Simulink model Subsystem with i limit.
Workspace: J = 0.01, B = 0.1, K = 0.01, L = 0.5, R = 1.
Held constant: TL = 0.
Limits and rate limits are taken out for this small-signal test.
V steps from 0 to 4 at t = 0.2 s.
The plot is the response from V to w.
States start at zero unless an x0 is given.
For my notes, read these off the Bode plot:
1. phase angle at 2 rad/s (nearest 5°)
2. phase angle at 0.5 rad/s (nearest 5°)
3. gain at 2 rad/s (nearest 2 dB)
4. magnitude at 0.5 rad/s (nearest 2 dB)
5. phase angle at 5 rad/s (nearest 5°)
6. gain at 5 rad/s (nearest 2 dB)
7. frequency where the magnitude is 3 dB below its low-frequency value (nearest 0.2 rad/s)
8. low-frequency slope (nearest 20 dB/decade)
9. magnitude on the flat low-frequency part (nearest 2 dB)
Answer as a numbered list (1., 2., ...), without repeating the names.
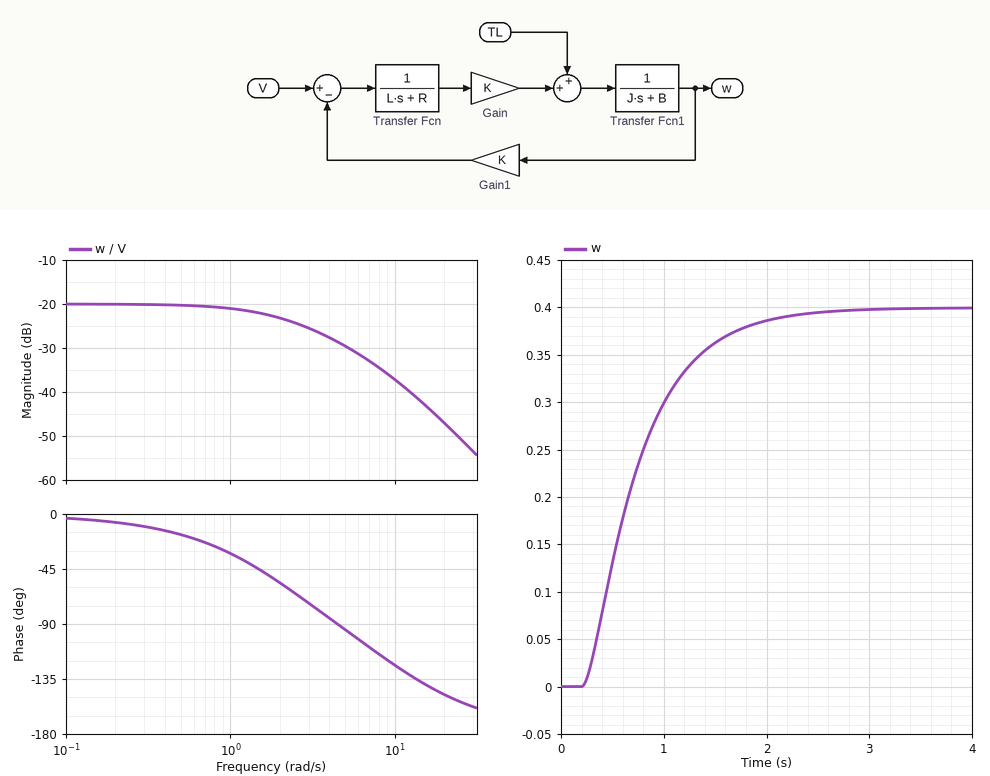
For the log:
1. -55°
2. -15°
3. -24 dB
4. -20 dB
5. -95°
6. -30 dB
7. 2.0 rad/s
8. 0 dB/decade
9. -20 dB
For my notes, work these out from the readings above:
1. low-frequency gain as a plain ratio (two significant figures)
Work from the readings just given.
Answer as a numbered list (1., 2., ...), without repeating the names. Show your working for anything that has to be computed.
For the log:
1. 10^(-20 / 20) = 0.10
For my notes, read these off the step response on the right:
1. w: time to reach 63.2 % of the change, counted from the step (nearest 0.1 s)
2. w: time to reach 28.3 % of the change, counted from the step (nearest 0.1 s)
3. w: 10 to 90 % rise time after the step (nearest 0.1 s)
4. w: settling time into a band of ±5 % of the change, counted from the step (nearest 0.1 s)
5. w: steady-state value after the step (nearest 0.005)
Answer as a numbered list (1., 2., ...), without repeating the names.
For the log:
1. 0.6 s
2. 0.3 s
3. 1.1 s
4. 1.6 s
5. 0.400
